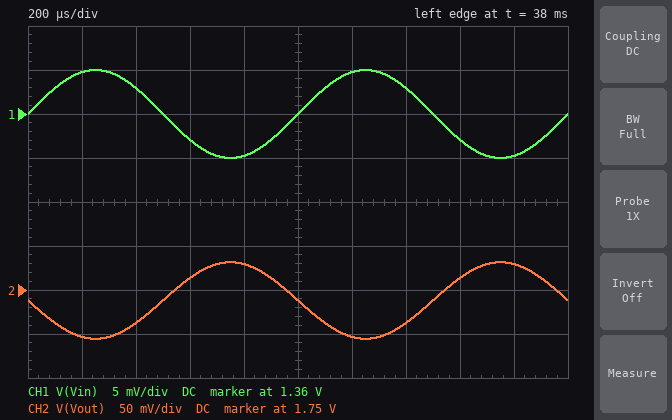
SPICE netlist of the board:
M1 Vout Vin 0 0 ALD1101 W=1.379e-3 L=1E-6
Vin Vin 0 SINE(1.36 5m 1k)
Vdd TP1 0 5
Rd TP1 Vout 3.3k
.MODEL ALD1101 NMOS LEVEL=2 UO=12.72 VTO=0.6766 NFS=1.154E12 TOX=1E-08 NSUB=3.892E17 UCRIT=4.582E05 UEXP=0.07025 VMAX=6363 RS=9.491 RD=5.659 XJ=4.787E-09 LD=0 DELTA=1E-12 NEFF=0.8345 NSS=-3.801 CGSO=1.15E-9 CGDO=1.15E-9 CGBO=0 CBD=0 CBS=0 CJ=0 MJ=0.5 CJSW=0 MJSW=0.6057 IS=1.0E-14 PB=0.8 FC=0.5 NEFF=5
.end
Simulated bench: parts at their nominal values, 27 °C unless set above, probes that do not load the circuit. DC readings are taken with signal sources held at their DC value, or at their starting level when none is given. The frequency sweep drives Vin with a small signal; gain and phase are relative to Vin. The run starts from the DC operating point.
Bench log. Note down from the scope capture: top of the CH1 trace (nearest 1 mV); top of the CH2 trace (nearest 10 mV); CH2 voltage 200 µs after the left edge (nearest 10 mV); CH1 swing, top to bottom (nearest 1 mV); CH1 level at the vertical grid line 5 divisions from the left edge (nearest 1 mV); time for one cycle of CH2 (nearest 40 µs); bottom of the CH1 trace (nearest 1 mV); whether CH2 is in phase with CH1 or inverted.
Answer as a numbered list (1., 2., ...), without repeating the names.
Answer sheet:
1. 1.365 V
2. 1.78 V
3. 1.70 V
4. 10 mV
5. 1.360 V
6. 1.00 ms
7. 1.355 V
8. inverted
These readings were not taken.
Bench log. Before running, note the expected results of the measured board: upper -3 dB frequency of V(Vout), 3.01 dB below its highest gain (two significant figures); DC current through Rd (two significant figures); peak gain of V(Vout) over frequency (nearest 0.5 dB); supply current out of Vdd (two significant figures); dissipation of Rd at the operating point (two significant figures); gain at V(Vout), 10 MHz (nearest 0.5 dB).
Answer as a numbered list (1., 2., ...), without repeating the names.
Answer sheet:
1. 32 MHz
2. 990 µA
3. 19.0 dB
4. 990 µA
5. 3.2 mW
6. 18.5 dB
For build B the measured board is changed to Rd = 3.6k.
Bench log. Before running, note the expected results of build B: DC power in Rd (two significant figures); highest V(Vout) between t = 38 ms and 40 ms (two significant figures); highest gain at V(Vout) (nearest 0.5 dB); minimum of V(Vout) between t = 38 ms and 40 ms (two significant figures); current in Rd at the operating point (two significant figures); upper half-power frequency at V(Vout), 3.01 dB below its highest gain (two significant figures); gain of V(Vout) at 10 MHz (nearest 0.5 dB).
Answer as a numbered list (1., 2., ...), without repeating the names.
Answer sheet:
1. 3.5 mW
2. 1.5 V
3. 19.5 dB
4. 1.4 V
5. 980 µA
6. 30 MHz
7. 19.0 dB
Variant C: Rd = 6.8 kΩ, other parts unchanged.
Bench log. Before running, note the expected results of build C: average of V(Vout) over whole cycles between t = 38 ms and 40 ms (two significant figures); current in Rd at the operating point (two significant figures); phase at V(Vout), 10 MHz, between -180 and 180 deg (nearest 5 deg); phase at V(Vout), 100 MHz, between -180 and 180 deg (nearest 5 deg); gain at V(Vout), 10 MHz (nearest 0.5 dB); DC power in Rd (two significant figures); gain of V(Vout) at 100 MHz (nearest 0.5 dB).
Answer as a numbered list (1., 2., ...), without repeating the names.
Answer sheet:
1. 230 mV
2. 700 µA
3. 165 deg
4. 75 deg
5. -6.0 dB
6. 3.3 mW
7. -2.0 dB
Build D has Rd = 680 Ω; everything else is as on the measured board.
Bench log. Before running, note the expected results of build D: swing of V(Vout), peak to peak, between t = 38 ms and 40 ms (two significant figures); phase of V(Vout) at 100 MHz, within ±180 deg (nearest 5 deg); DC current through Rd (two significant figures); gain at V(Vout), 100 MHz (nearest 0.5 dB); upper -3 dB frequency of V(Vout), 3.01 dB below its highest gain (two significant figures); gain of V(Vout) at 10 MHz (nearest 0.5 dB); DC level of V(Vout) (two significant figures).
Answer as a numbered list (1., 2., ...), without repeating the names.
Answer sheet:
1. 19 mV
2. 125 deg
3. 1.0 mA
4. 4.5 dB
5. 250 MHz
6. 5.5 dB
7. 4.3 V
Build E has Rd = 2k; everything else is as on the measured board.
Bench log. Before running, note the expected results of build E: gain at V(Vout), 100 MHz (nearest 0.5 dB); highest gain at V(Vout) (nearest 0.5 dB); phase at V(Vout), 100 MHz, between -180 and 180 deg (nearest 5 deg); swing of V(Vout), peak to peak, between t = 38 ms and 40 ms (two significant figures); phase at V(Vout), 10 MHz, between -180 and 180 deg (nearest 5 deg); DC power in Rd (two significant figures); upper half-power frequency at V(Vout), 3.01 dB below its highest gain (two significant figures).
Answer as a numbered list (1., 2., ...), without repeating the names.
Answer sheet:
1. 8.5 dB
2. 15.0 dB
3. 95 deg
4. 55 mV
5. 165 deg
6. 2.0 mW
7. 53 MHz
